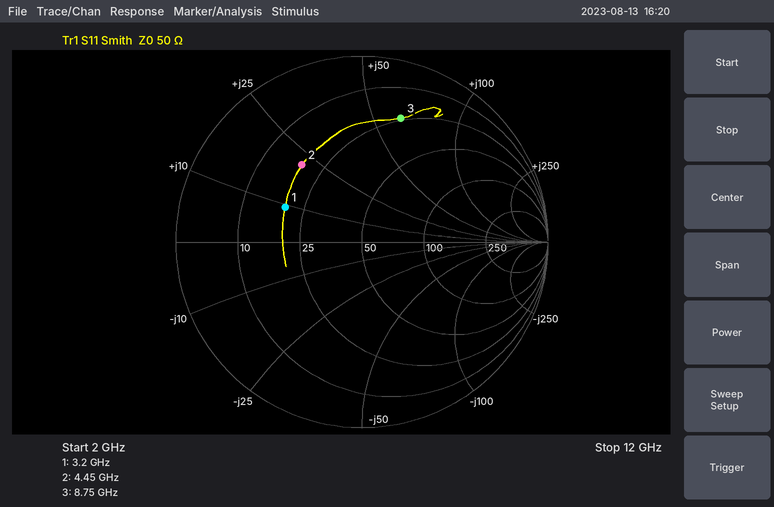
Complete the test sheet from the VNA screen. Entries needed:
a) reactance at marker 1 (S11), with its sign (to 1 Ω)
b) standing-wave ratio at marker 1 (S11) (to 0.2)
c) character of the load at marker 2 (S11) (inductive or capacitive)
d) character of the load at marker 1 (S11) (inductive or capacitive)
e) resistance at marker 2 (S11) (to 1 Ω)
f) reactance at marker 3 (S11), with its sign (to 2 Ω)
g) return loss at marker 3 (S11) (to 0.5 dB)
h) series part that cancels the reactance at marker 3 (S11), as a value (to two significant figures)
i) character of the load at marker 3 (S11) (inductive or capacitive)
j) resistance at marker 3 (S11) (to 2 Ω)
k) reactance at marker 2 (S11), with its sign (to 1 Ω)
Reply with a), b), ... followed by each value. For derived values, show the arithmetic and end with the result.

a) +9 Ω
b) 2.6
c) inductive
d) inductive
e) 19 Ω
f) +62 Ω
g) 3.0 dB
h) C = 1/(2π × 8.75 GHz × 62 Ω) ≈ 293 fF, so 290 fF to two significant figures
i) inductive
j) 24 Ω
k) +22 Ω
